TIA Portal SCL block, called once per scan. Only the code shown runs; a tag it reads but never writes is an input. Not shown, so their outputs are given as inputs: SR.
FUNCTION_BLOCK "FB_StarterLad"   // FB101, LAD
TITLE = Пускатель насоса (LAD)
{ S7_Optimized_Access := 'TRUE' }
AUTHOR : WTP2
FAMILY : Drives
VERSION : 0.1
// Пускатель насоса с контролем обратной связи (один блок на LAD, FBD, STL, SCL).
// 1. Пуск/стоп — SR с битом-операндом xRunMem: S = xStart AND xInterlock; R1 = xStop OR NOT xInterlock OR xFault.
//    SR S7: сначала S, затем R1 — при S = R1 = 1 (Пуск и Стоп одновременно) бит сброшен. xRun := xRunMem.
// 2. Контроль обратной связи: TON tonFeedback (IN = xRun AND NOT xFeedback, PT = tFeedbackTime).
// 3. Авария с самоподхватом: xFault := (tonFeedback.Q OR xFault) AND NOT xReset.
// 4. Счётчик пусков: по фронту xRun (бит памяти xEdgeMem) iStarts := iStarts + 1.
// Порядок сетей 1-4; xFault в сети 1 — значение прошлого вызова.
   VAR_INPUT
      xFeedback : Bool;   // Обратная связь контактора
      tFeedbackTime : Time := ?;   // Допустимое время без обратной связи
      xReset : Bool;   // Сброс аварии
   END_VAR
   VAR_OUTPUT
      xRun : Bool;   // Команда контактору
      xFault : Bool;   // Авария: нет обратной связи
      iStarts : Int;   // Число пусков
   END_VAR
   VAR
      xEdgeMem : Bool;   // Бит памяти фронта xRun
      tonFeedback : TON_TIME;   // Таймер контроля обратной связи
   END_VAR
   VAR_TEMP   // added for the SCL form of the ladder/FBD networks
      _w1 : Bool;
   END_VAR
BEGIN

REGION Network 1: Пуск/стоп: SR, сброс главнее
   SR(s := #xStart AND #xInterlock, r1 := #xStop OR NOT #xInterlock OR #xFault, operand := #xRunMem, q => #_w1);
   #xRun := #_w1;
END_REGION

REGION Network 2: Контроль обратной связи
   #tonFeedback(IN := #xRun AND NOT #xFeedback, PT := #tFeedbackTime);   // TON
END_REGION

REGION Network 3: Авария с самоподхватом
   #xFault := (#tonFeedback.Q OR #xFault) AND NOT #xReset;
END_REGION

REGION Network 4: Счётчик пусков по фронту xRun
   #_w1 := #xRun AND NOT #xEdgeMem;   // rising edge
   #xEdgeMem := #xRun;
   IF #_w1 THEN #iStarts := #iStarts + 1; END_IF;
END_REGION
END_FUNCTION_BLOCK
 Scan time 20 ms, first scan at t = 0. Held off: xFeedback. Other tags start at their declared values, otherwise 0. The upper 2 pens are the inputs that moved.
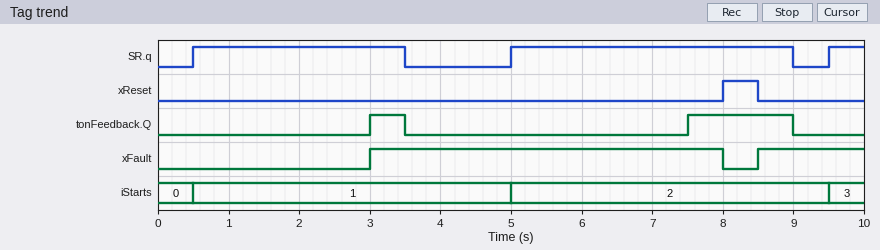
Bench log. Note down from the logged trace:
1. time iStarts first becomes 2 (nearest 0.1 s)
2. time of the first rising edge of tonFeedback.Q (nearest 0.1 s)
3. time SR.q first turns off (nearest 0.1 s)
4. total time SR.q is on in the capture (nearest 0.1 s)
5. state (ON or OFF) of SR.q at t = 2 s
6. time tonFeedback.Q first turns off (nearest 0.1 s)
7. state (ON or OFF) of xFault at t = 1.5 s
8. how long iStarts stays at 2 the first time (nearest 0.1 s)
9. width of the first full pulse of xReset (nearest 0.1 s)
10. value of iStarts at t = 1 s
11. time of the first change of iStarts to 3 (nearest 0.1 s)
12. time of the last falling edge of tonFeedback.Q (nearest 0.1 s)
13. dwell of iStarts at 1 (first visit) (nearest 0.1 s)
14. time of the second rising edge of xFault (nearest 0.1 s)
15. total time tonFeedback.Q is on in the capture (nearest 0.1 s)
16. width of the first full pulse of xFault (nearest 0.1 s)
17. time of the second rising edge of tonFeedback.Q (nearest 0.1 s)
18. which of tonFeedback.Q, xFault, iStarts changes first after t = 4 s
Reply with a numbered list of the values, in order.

1. 5.0 s
2. 3.0 s
3. 3.5 s
4. 7.5 s
5. ON
6. 3.5 s
7. OFF
8. 4.5 s
9. 0.5 s
10. 1
11. 9.5 s
12. 9.0 s
13. 4.5 s
14. 8.5 s
15. 2.0 s
16. 5.0 s
17. 7.5 s
18. iStarts
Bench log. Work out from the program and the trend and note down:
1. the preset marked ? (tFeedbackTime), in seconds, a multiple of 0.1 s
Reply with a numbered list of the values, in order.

1. 2.5 s
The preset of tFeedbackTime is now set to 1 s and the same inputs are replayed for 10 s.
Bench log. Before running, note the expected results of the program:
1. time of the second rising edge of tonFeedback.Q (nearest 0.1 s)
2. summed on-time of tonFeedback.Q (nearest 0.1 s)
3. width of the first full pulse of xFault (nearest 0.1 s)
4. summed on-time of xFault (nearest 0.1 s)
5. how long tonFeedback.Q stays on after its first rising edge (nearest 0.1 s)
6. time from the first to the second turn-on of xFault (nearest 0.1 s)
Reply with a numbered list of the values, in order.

1. 6.0 s
2. 5.0 s
3. 6.5 s
4. 8.0 s
5. 2.0 s
6. 7.0 s
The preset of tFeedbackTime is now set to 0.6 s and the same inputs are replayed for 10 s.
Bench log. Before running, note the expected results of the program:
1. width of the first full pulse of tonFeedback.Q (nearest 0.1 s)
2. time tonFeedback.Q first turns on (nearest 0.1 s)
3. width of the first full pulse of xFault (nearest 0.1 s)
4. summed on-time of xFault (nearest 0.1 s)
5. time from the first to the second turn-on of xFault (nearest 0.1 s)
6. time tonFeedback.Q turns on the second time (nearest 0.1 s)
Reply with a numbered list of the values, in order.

1. 2.4 s
2. 1.1 s
3. 6.9 s
4. 8.4 s
5. 7.4 s
6. 5.6 s
